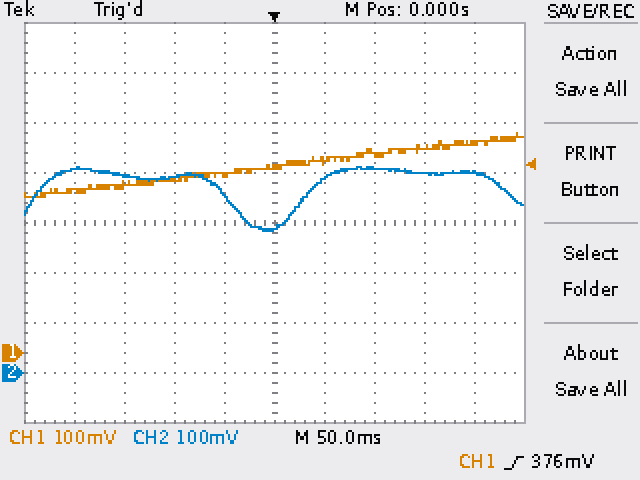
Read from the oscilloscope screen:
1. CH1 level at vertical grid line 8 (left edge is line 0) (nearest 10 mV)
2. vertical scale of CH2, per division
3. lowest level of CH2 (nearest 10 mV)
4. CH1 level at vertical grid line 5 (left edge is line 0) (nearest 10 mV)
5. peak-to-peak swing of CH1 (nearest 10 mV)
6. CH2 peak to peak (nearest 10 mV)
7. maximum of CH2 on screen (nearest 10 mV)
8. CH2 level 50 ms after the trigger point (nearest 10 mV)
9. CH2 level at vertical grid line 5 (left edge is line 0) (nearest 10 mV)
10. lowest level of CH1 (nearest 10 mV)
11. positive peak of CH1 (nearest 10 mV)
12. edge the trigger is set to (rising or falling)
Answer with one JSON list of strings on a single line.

["410 mV", "100 mV", "280 mV", "370 mV", "130 mV", "130 mV", "410 mV", "390 mV", "290 mV", "310 mV", "440 mV", "rising"]
